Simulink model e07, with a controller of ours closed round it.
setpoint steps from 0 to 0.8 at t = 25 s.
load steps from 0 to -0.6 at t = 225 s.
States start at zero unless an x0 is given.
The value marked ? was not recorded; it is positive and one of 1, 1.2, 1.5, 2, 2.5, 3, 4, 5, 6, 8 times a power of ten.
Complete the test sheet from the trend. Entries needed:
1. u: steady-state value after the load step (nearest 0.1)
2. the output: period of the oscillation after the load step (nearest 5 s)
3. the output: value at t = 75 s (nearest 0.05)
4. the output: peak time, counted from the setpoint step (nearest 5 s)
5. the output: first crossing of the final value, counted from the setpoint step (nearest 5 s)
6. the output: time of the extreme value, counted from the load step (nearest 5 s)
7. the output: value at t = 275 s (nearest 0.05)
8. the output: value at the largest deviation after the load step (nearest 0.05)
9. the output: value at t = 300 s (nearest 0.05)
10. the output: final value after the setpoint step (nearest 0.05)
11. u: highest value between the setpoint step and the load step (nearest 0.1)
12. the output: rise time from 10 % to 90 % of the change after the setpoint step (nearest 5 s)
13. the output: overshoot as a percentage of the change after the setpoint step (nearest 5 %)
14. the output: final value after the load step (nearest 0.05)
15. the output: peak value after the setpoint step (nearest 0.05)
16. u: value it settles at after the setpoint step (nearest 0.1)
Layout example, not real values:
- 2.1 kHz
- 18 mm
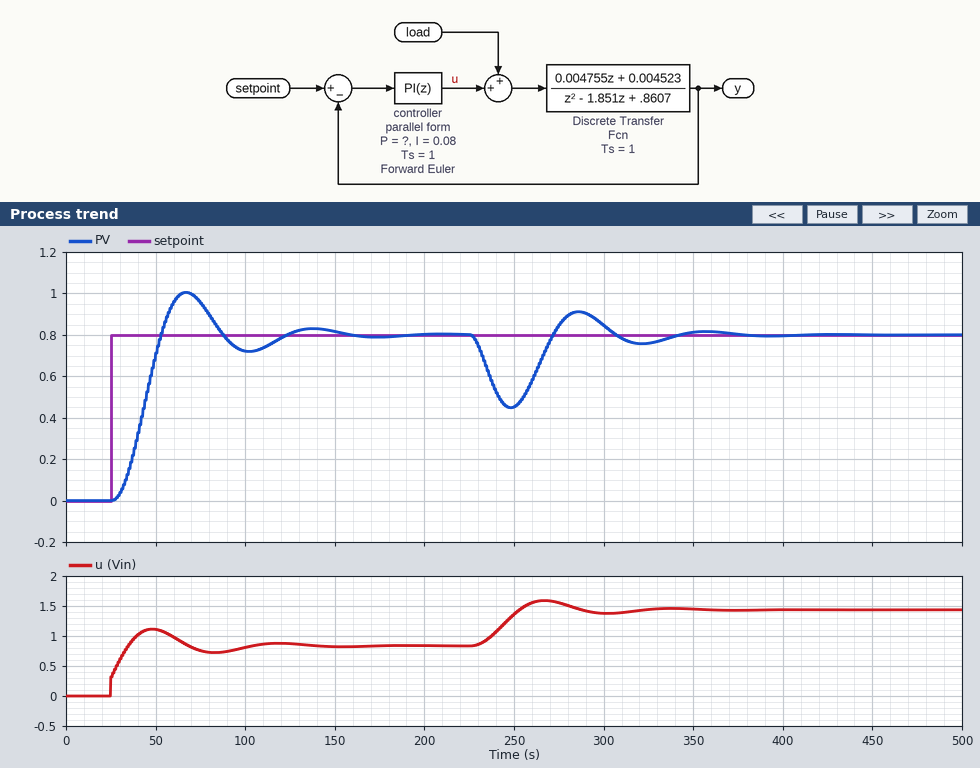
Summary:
- 1.4
- 75 s
- 0.95
- 40 s
- 30 s
- 25 s
- 0.85
- 0.45
- 0.85
- 0.80
- 1.1
- 20 s
- 25 %
- 0.80
- 1.00
- 0.8
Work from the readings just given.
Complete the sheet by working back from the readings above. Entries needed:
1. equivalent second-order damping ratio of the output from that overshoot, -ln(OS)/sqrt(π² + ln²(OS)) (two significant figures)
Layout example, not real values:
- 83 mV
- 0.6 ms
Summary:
- 0.40
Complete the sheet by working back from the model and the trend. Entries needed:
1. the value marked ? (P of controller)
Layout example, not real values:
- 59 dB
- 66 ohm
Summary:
- 0.4
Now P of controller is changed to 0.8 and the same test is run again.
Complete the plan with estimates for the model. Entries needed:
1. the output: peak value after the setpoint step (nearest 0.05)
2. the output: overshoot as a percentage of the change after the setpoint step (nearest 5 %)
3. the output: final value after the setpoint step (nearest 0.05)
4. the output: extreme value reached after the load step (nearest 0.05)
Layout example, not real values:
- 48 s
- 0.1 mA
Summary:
- 0.90
- 15 %
- 0.80
- 0.50
